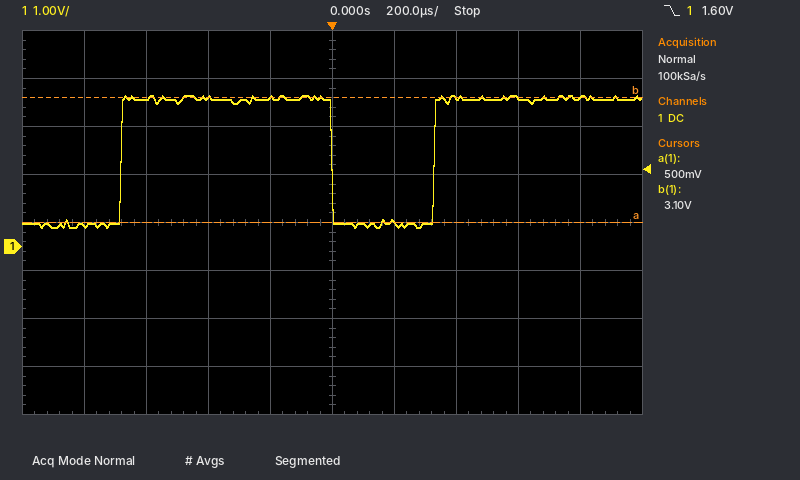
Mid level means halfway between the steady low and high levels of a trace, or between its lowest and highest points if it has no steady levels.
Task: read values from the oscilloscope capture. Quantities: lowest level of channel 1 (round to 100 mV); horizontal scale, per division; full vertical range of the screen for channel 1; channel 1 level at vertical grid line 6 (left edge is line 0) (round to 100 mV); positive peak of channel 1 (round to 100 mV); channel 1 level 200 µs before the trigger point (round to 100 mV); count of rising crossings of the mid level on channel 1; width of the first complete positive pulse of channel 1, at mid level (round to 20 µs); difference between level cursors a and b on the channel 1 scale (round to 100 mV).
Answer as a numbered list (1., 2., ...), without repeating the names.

1. 400 mV
2. 200 µs
3. 8 V
4. 500 mV
5. 3.1 V
6. 3.1 V
7. 2
8. 680 µs
9. 2.6 V
